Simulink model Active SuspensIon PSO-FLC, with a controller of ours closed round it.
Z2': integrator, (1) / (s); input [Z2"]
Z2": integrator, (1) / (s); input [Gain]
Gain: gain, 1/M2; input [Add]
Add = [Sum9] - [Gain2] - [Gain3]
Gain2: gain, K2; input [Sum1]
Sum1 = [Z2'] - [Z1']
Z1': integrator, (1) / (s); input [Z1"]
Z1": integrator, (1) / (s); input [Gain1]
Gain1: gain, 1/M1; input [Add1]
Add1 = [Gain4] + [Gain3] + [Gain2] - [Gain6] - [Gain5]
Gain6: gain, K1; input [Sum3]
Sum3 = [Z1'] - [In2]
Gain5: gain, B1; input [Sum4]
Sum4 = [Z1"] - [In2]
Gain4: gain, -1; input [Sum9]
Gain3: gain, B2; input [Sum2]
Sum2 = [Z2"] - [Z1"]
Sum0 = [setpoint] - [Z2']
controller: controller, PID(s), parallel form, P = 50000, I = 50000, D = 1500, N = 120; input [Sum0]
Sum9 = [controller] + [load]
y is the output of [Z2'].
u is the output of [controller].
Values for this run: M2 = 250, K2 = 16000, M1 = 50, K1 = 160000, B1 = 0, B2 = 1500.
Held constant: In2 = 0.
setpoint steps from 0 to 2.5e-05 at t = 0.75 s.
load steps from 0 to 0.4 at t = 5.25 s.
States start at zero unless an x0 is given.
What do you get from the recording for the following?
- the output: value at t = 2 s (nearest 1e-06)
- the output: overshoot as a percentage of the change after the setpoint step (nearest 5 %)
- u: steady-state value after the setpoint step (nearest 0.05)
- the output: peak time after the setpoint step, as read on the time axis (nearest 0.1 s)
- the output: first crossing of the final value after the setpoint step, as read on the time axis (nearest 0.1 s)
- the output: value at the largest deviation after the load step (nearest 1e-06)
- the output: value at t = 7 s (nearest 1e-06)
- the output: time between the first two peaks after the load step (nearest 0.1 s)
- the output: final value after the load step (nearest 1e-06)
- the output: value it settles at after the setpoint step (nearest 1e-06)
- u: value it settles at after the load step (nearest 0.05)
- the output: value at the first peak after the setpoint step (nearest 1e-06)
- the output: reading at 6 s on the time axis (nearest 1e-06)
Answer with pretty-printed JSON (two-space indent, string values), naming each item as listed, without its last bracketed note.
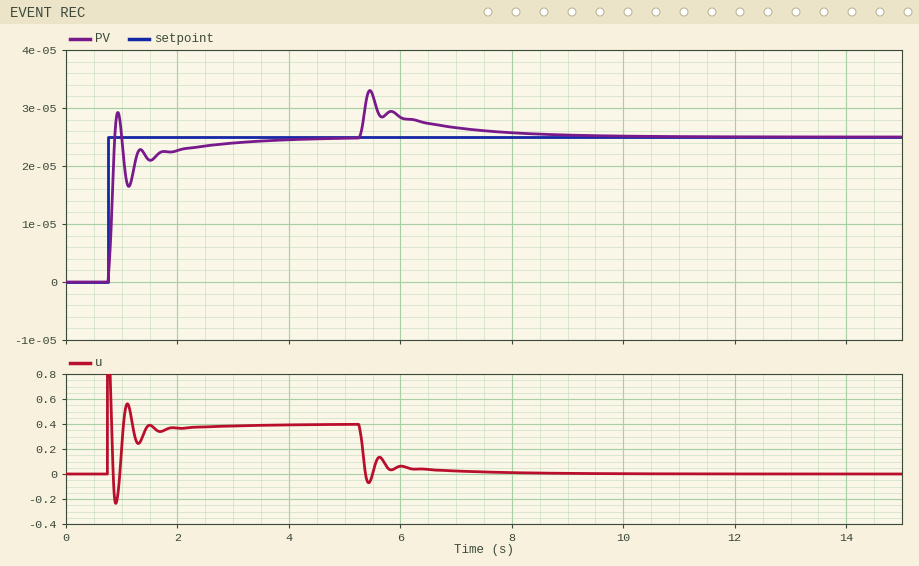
{
  "the output: value at t = 2 s": "0.000023",
  "the output: overshoot as a percentage of the change after the setpoint step": "15 %",
  "u: steady-state value after the setpoint step": "0.40",
  "the output: peak time after the setpoint step, as read on the time axis": "0.9 s",
  "the output: first crossing of the final value after the setpoint step, as read on the time axis": "0.9 s",
  "the output: value at the largest deviation after the load step": "0.000033",
  "the output: value at t = 7 s": "0.000027",
  "the output: time between the first two peaks after the load step": "0.4 s",
  "the output: final value after the load step": "0.000025",
  "the output: value it settles at after the setpoint step": "0.000025",
  "u: value it settles at after the load step": "0.00",
  "the output: value at the first peak after the setpoint step": "0.000029",
  "the output: reading at 6 s on the time axis": "0.000028"
}
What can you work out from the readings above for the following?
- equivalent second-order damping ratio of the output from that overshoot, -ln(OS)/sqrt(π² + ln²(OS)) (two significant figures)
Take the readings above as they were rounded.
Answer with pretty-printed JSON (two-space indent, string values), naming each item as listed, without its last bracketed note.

{
  "equivalent second-order damping ratio of the output from that overshoot, -ln(OS)/sqrt(π² + ln²(OS))": "0.52"
}
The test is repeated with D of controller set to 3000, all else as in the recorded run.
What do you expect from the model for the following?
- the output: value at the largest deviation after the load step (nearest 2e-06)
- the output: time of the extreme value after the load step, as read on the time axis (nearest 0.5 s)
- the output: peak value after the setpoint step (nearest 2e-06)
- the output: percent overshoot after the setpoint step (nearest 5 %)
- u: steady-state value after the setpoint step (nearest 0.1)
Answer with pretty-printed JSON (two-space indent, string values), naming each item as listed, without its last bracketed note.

{
  "the output: value at the largest deviation after the load step": "0.000032",
  "the output: time of the extreme value after the load step, as read on the time axis": "5.5 s",
  "the output: peak value after the setpoint step": "0.000028",
  "the output: percent overshoot after the setpoint step": "10 %",
  "u: steady-state value after the setpoint step": "0.4"
}
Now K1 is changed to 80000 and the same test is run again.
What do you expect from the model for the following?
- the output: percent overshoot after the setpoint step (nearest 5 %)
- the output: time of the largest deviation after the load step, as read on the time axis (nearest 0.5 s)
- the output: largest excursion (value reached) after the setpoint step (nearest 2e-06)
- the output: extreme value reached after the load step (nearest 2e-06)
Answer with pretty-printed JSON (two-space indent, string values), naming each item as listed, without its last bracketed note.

{
  "the output: percent overshoot after the setpoint step": "30 %",
  "the output: time of the largest deviation after the load step, as read on the time axis": "5.5 s",
  "the output: largest excursion (value reached) after the setpoint step": "0.000032",
  "the output: extreme value reached after the load step": "0.000034"
}
